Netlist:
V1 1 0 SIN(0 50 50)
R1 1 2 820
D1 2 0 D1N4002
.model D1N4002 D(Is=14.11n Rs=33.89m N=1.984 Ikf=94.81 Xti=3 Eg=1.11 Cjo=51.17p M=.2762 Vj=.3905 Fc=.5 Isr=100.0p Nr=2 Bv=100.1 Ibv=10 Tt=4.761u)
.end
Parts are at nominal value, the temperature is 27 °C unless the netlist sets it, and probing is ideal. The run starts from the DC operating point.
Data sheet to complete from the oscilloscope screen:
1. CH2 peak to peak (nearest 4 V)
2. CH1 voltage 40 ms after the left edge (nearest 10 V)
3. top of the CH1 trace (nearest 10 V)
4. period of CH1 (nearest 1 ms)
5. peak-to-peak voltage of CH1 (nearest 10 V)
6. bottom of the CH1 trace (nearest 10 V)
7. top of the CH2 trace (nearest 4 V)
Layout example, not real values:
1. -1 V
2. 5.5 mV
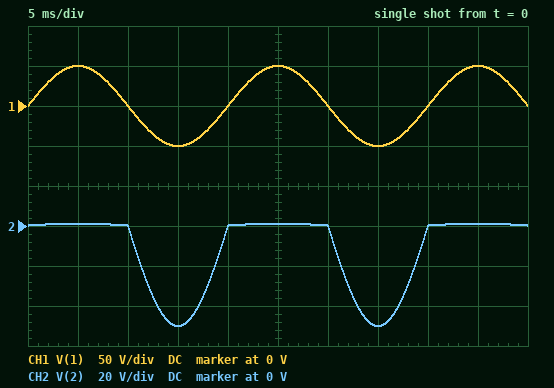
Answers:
1. 52 V
2. 0 V
3. 50 V
4. 20 ms
5. 100 V
6. -50 V
7. 0 V
